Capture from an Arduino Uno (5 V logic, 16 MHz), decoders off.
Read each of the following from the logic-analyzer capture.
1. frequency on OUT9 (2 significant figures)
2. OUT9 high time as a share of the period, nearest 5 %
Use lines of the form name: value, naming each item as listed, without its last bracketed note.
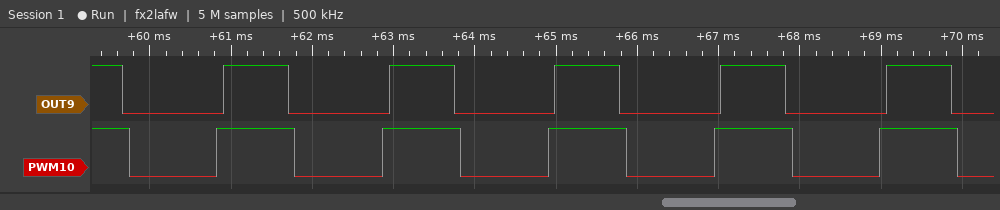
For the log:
frequency on OUT9: 490 Hz
OUT9 high time as a share of the period, nearest 5 %: 40 %
